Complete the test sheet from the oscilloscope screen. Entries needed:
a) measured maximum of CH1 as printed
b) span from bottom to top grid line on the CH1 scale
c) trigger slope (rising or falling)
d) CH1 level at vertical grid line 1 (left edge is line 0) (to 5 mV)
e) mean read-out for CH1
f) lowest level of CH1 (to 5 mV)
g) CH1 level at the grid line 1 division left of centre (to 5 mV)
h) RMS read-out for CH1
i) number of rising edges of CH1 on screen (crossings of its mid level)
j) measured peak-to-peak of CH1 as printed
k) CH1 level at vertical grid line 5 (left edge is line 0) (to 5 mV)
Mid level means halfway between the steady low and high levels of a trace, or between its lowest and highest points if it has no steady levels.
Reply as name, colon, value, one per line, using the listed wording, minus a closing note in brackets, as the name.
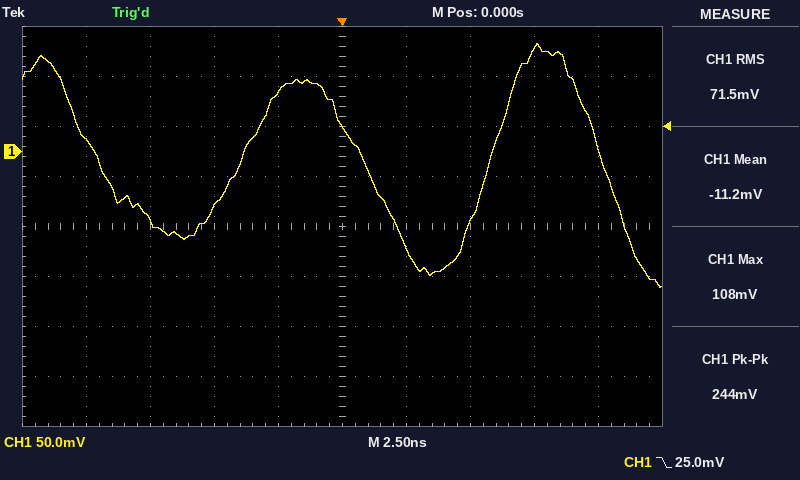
measured maximum of CH1 as printed: 108 mV
span from bottom to top grid line on the CH1 scale: 400 mV
trigger slope: falling
CH1 level at vertical grid line 1 (left edge is line 0): 10 mV
mean read-out for CH1: -11.2 mV
lowest level of CH1: -135 mV
CH1 level at the grid line 1 division left of centre: 60 mV
RMS read-out for CH1: 71.5 mV
number of rising edges of CH1 on screen: 2
measured peak-to-peak of CH1 as printed: 244 mV
CH1 level at vertical grid line 5 (left edge is line 0): 25 mV
